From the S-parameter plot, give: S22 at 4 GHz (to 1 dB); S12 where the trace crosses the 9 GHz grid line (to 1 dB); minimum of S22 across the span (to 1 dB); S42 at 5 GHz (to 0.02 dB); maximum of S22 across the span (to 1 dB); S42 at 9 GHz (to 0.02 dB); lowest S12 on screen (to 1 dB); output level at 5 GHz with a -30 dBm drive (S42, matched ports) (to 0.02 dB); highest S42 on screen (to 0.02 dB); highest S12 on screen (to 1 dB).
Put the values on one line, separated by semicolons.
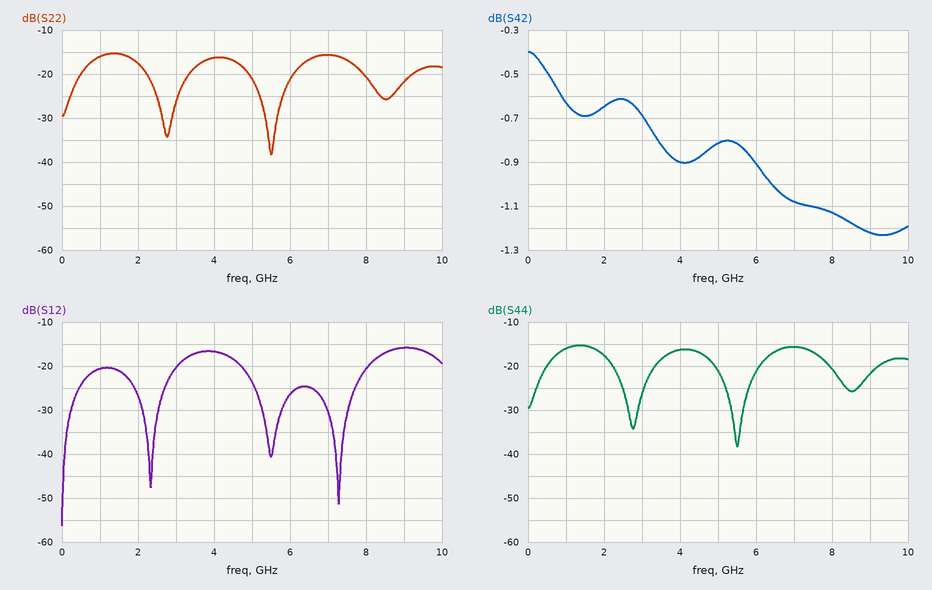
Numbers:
-16 dB; -16 dB; -38 dB; -0.82 dB; -15 dB; -1.22 dB; -56 dB; -30.82 dBm; -0.40 dB; -16 dB
